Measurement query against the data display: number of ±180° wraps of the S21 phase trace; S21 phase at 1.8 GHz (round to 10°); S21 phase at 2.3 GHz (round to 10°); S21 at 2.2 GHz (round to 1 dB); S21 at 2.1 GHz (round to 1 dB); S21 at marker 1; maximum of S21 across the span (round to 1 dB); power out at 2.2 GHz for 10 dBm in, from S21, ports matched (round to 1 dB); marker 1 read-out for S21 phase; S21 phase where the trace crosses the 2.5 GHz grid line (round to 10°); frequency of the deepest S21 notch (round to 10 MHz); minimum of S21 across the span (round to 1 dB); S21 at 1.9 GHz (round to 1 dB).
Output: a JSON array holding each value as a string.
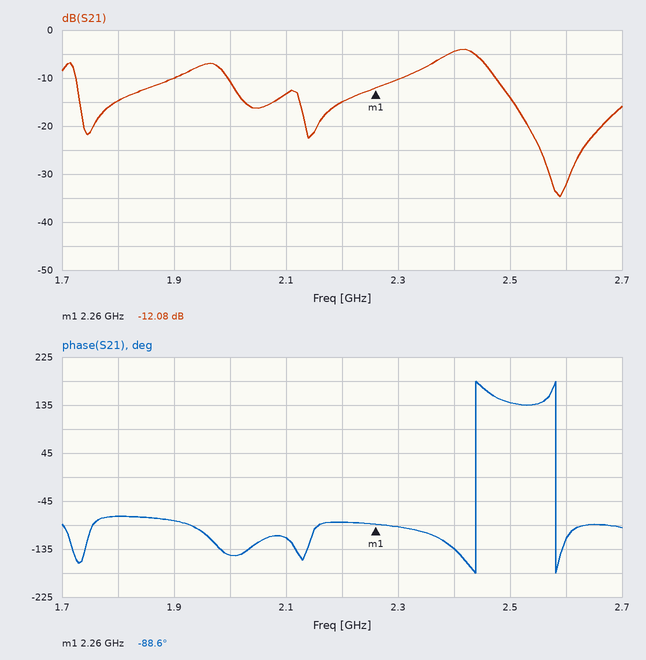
["2", "-70°", "-90°", "-15 dB", "-13 dB", "-12.08 dB", "-4 dB", "-5 dBm", "-88.6°", "140°", "2.59 GHz", "-35 dB", "-10 dB"]
